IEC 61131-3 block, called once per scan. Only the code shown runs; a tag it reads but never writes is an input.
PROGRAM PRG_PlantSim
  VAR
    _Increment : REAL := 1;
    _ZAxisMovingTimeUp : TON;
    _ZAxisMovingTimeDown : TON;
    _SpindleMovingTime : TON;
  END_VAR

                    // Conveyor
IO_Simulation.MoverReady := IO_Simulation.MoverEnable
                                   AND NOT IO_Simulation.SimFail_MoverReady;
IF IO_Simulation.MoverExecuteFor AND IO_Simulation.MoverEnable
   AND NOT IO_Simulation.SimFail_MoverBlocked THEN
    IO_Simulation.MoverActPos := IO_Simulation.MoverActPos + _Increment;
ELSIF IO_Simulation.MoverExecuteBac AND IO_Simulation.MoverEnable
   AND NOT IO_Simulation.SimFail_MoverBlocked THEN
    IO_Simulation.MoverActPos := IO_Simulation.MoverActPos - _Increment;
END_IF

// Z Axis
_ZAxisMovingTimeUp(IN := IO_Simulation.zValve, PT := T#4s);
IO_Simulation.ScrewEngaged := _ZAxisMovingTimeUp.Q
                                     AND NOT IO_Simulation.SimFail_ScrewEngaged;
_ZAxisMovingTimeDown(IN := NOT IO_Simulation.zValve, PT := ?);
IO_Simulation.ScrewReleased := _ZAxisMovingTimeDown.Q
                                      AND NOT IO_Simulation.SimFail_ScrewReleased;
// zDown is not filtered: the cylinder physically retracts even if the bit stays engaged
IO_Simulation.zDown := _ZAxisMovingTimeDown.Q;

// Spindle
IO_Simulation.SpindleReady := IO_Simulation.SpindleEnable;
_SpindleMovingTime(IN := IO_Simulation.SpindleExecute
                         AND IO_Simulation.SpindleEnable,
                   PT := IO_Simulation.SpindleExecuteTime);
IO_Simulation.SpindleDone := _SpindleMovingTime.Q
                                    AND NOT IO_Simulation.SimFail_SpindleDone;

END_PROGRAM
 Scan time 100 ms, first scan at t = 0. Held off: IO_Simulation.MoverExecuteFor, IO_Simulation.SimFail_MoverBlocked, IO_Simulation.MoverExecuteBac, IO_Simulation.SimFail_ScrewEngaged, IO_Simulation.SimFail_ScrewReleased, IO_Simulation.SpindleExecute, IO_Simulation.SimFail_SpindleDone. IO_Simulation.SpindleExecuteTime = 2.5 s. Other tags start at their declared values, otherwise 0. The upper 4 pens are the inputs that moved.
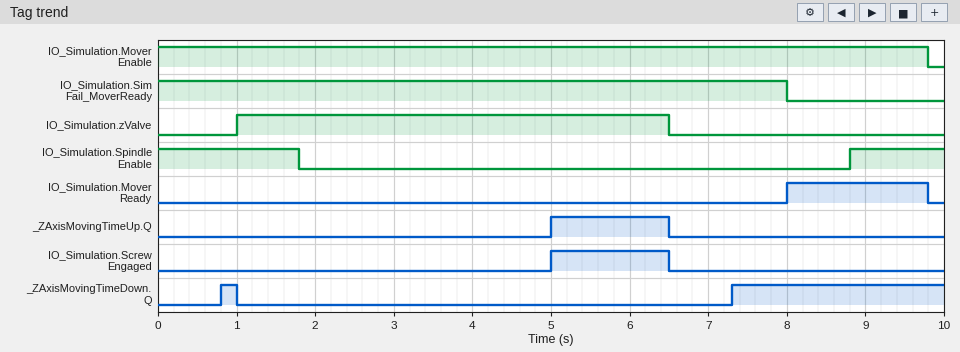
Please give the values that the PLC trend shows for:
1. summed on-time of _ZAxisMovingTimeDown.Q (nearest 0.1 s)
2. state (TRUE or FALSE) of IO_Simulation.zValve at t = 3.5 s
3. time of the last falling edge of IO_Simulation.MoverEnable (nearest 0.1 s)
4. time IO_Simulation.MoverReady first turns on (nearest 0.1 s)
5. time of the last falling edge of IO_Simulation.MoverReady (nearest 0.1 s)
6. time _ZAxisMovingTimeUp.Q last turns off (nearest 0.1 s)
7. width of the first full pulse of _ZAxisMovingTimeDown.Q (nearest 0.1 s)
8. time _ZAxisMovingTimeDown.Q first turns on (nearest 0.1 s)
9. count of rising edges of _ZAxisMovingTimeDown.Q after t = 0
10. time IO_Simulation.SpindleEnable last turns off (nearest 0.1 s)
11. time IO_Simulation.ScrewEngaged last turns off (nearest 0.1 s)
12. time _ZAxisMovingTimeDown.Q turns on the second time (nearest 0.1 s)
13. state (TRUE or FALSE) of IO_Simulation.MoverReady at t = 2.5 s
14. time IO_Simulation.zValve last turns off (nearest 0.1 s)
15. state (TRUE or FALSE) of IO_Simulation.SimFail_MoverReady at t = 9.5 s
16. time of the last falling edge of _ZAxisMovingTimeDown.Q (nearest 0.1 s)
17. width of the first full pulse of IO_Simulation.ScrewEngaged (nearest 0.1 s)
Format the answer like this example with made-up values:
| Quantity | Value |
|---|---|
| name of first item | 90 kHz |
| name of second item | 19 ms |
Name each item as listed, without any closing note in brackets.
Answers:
| Quantity | Value |
|---|---|
| summed on-time of _ZAxisMovingTimeDown.Q | 2.9 s |
| state (TRUE or FALSE) of IO_Simulation.zValve at t = 3.5 s | TRUE |
| time of the last falling edge of IO_Simulation.MoverEnable | 9.8 s |
| time IO_Simulation.MoverReady first turns on | 8.0 s |
| time of the last falling edge of IO_Simulation.MoverReady | 9.8 s |
| time _ZAxisMovingTimeUp.Q last turns off | 6.5 s |
| width of the first full pulse of _ZAxisMovingTimeDown.Q | 0.2 s |
| time _ZAxisMovingTimeDown.Q first turns on | 0.8 s |
| count of rising edges of _ZAxisMovingTimeDown.Q after t = 0 | 2 |
| time IO_Simulation.SpindleEnable last turns off | 1.8 s |
| time IO_Simulation.ScrewEngaged last turns off | 6.5 s |
| time _ZAxisMovingTimeDown.Q turns on the second time | 7.3 s |
| state (TRUE or FALSE) of IO_Simulation.MoverReady at t = 2.5 s | FALSE |
| time IO_Simulation.zValve last turns off | 6.5 s |
| state (TRUE or FALSE) of IO_Simulation.SimFail_MoverReady at t = 9.5 s | FALSE |
| time of the last falling edge of _ZAxisMovingTimeDown.Q | 1.0 s |
| width of the first full pulse of IO_Simulation.ScrewEngaged | 1.5 s |
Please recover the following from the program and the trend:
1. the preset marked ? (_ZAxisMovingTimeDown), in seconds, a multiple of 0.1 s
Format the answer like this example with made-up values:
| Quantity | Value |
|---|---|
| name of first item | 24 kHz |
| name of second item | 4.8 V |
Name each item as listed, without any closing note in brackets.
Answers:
| Quantity | Value |
|---|---|
| the preset marked ? (_ZAxisMovingTimeDown), in seconds, a multiple of 0.1 s | 0.8 s |
